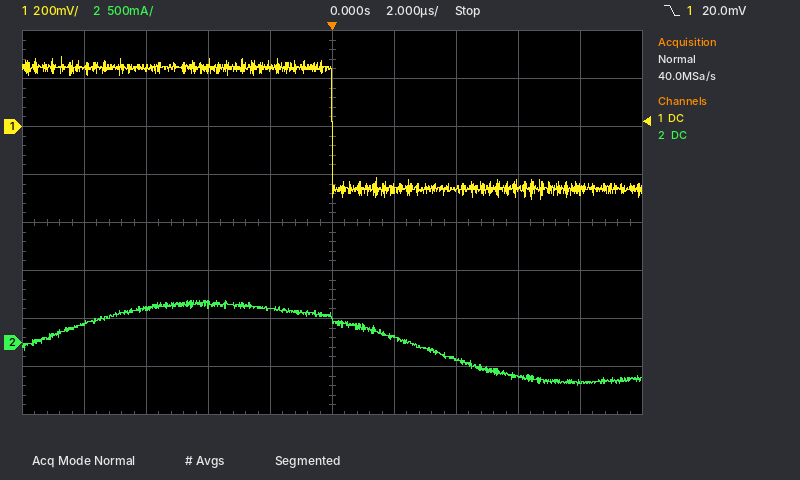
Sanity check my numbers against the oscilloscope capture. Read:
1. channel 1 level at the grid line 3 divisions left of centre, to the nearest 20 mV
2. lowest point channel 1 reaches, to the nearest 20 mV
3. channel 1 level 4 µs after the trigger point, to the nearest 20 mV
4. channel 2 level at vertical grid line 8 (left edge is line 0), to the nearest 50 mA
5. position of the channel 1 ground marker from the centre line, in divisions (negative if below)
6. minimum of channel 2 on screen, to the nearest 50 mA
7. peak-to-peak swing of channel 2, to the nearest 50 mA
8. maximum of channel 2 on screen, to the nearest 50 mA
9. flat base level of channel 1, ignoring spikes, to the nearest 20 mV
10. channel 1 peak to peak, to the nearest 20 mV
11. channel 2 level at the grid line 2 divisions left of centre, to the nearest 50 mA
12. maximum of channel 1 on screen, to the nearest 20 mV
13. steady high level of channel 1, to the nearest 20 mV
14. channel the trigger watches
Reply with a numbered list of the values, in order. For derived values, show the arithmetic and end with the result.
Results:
1. 240 mV
2. -300 mV
3. -260 mV
4. -350 mA
5. +2.0 div
6. -450 mA
7. 450 mA − (-450 mA) = 900 mA
8. 450 mA
9. -260 mV
10. 300 mV − (-300 mV) = 600 mV
11. 400 mA
12. 300 mV
13. 240 mV
14. channel 1
